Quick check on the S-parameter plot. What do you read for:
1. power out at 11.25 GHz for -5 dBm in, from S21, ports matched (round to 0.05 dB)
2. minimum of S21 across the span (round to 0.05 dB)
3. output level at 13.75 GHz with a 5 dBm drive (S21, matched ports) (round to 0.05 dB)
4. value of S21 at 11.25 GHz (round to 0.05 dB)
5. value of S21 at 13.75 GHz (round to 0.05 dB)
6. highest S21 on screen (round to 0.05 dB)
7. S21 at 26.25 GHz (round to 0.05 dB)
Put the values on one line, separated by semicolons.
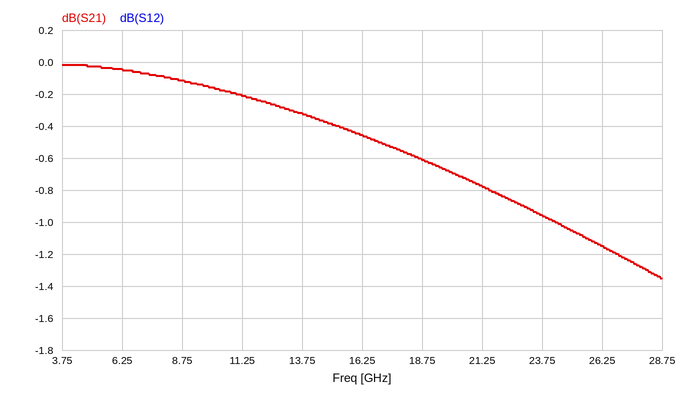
-5.20 dBm; -1.35 dB; 4.70 dBm; -0.20 dB; -0.30 dB; 0.00 dB; -1.15 dB
